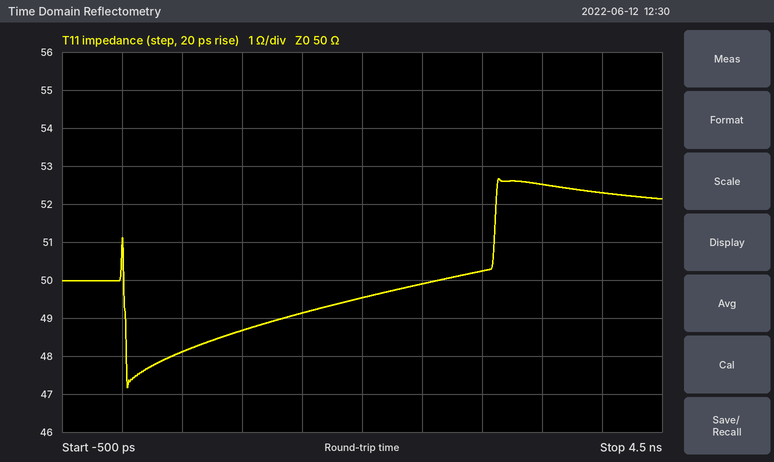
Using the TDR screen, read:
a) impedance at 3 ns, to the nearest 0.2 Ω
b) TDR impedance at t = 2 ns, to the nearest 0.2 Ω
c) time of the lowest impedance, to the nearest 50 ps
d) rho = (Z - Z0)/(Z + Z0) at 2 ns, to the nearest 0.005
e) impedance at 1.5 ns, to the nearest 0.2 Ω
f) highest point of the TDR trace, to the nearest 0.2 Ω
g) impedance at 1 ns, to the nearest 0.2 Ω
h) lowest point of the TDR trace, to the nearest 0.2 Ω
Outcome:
50.2 Ω
49.6 Ω
50 ps
-0.005
49.2 Ω
52.6 Ω
48.6 Ω
47.2 Ω
